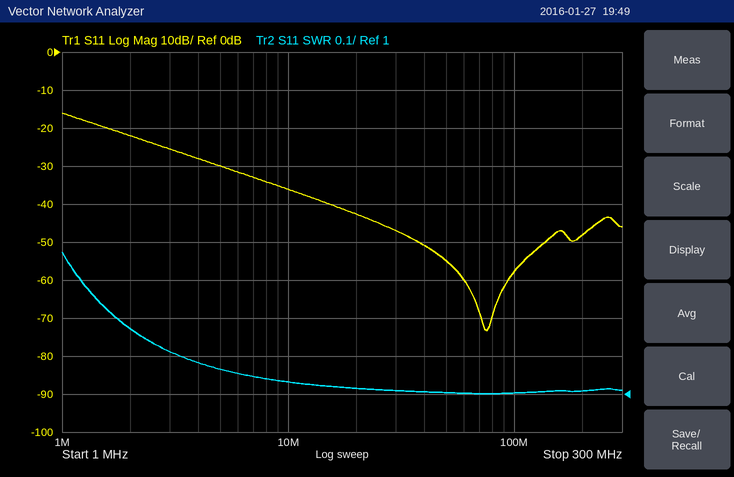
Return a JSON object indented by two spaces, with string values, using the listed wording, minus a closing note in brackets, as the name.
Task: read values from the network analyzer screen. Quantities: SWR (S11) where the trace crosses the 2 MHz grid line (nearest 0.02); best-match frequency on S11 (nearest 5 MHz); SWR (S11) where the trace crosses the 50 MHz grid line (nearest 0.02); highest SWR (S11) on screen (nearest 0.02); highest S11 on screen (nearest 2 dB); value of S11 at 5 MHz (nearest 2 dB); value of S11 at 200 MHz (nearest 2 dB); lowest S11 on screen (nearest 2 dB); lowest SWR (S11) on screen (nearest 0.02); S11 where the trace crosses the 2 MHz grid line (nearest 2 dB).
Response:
{
  "SWR (S11) where the trace crosses the 2 MHz grid line": "1.18",
  "best-match frequency on S11": "75 MHz",
  "SWR (S11) where the trace crosses the 50 MHz grid line": "1.00",
  "highest SWR (S11) on screen": "1.38",
  "highest S11 on screen": "-16 dB",
  "value of S11 at 5 MHz": "-30 dB",
  "value of S11 at 200 MHz": "-48 dB",
  "lowest S11 on screen": "-74 dB",
  "lowest SWR (S11) on screen": "1.00",
  "S11 where the trace crosses the 2 MHz grid line": "-22 dB"
}
